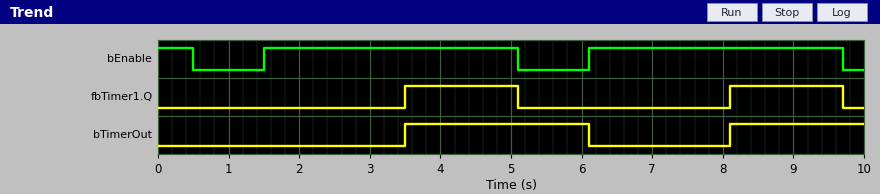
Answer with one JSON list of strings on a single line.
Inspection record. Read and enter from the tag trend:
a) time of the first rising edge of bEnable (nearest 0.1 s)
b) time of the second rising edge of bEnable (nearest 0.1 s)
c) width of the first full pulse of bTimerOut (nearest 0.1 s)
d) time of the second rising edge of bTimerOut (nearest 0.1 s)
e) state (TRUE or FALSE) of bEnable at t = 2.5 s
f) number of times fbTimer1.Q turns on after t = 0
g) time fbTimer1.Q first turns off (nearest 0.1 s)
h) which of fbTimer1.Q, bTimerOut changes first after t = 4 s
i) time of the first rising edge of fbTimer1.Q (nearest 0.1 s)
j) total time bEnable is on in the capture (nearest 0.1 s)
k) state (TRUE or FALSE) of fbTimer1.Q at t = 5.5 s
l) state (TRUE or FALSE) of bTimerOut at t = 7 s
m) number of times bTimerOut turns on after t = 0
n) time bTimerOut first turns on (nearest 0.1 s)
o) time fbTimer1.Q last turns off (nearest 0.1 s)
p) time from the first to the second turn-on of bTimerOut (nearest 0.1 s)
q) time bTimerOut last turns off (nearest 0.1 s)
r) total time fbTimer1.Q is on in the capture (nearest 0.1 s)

["1.5 s", "6.1 s", "2.6 s", "8.1 s", "TRUE", "2", "5.1 s", "fbTimer1.Q", "3.5 s", "7.7 s", "FALSE", "FALSE", "2", "3.5 s", "9.7 s", "4.6 s", "6.1 s", "3.2 s"]
